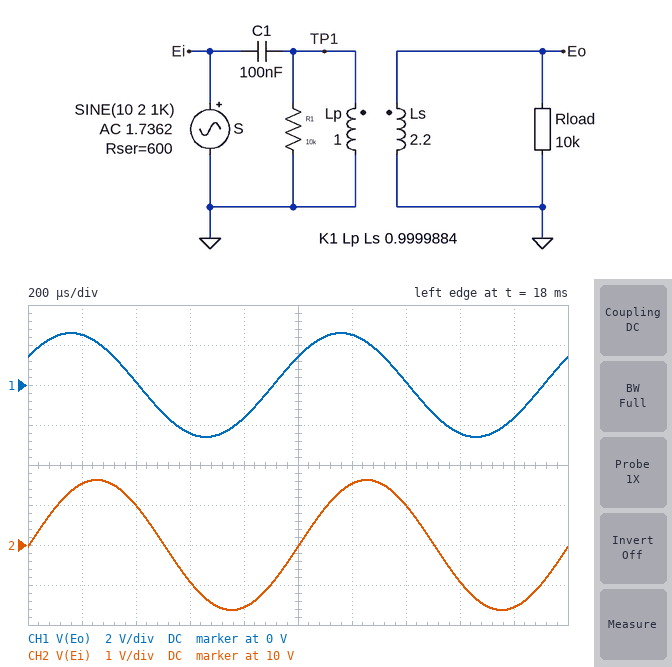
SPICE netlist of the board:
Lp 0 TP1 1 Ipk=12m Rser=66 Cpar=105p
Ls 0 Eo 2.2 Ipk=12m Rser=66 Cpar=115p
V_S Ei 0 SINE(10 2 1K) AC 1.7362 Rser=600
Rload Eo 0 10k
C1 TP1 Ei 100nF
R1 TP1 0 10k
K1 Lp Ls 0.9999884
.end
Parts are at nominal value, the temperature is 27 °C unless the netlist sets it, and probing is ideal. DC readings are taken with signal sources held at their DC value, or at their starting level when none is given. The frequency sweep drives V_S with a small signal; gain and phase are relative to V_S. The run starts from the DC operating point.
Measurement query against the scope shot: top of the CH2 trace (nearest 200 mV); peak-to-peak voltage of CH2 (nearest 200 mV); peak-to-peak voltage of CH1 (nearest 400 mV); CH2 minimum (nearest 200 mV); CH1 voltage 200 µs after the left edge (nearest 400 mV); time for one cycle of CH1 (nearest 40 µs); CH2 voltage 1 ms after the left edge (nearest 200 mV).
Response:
11.6 V
3.2 V
5.2 V
8.4 V
2.4 V
1.00 ms
10.0 V
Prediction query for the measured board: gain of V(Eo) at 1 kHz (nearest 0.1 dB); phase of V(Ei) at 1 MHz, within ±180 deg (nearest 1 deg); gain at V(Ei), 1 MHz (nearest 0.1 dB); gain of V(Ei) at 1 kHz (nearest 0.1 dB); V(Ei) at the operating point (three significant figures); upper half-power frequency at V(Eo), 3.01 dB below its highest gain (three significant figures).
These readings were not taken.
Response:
2.3 dB
-45 deg
-6.5 dB
-1.8 dB
10.0 V
829 kHz
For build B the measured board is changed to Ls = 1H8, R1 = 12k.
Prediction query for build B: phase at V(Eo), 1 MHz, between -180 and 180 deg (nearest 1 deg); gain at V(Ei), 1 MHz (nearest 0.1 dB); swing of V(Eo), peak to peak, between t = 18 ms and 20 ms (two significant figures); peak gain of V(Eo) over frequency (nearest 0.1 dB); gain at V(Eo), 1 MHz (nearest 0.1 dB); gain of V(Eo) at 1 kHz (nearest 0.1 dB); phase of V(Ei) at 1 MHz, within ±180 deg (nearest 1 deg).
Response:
-54 deg
-5.4 dB
5.0 V
2.6 dB
-1.4 dB
2.0 dB
-43 deg
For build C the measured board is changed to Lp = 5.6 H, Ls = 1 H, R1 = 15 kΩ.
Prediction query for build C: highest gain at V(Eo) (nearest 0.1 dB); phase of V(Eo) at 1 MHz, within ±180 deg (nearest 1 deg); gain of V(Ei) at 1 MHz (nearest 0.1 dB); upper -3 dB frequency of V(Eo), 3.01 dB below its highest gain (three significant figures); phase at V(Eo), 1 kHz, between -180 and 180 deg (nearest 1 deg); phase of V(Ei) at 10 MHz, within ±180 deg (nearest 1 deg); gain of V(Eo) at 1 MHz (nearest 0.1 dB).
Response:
-1.9 dB
-29 deg
-1.3 dB
3.62 MHz
9 deg
-75 deg
-7.9 dB
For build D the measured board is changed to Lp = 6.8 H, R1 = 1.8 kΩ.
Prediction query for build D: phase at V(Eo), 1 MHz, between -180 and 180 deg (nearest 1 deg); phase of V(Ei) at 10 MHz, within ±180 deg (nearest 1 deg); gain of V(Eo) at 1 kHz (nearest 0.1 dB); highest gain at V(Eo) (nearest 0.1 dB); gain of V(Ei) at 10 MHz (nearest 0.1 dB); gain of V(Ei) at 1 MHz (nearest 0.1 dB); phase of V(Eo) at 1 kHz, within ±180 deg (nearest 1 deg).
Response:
-29 deg
-71 deg
-9.2 dB
-0.1 dB
-12.3 dB
-3.5 dB
36 deg
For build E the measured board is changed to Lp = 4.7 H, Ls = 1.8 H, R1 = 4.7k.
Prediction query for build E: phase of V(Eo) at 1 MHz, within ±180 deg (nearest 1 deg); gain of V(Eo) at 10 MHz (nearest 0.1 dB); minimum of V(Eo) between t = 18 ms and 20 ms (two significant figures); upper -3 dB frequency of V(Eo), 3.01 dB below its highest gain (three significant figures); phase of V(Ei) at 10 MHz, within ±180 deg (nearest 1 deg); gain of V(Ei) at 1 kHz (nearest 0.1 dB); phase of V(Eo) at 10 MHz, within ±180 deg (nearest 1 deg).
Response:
-33 deg
-41.4 dB
-1.0 V
2.86 MHz
-74 deg
-1.2 dB
109 deg
